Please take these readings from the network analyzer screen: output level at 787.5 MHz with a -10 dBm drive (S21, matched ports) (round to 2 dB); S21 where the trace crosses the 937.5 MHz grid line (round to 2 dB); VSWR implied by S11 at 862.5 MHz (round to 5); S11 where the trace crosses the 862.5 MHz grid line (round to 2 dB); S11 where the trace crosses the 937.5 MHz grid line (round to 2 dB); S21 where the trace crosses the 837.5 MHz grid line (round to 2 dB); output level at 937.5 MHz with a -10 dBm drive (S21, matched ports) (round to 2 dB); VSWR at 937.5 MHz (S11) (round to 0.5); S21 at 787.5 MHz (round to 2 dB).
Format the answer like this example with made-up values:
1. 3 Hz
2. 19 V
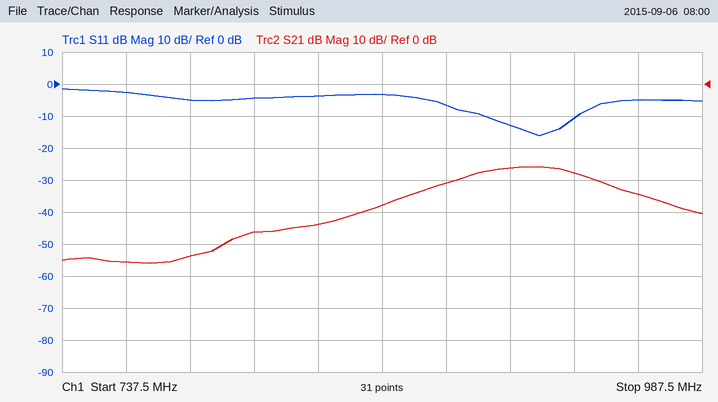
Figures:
1. -64 dBm
2. -28 dB
3. 5
4. -4 dB
5. -10 dB
6. -44 dB
7. -38 dBm
8. 2.0
9. -54 dB
